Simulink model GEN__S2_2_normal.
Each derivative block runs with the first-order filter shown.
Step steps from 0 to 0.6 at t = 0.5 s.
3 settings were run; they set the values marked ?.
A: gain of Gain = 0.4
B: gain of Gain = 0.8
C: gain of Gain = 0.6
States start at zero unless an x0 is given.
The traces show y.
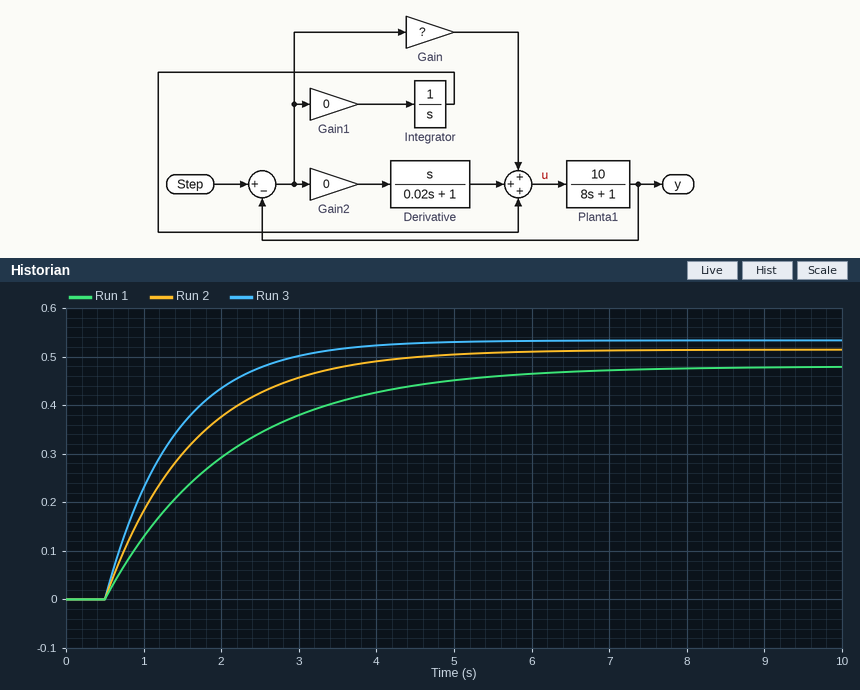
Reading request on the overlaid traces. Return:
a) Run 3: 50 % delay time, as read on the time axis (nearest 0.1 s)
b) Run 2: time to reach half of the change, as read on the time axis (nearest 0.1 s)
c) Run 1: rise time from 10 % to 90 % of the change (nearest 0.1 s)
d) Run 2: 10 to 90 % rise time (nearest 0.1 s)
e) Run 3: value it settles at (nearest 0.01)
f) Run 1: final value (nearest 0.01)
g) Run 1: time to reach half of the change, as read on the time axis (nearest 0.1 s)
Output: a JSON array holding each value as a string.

["1.1 s", "1.3 s", "3.5 s", "2.5 s", "0.53", "0.48", "1.6 s"]
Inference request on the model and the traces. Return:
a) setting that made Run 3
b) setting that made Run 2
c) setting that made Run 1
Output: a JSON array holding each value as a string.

["B", "C", "A"]
